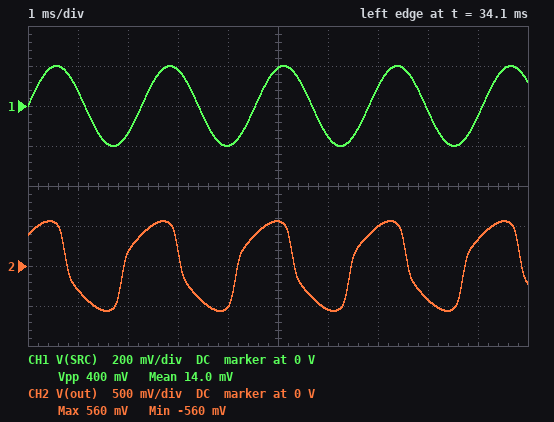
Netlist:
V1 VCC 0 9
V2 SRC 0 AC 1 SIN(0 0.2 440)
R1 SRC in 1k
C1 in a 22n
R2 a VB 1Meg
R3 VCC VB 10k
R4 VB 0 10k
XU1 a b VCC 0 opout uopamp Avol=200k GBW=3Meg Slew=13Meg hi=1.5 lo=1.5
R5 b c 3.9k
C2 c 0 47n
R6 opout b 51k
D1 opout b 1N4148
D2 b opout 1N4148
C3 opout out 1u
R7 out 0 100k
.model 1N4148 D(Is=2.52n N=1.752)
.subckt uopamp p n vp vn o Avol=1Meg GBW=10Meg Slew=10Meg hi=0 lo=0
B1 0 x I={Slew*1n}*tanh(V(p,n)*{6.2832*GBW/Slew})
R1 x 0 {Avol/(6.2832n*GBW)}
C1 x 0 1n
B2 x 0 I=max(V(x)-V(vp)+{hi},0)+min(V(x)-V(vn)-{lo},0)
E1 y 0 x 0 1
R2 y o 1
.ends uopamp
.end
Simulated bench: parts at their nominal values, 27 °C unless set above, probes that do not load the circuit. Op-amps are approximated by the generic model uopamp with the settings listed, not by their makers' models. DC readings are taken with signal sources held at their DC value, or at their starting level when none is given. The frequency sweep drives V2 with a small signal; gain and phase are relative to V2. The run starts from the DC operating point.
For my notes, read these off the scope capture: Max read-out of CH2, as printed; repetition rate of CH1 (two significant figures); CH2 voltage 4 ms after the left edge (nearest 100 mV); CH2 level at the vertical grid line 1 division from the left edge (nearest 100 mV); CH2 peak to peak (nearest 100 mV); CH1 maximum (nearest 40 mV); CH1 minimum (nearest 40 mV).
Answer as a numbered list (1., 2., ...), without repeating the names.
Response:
1. 560 mV
2. 440 Hz
3. -500 mV
4. -300 mV
5. 1.1 V
6. 200 mV
7. -200 mV
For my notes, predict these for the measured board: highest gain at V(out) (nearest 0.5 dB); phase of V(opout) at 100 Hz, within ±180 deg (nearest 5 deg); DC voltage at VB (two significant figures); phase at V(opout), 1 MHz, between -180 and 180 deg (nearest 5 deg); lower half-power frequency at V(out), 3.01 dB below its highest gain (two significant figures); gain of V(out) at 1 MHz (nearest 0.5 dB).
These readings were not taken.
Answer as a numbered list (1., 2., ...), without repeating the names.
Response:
1. 23.0 dB
2. 55 deg
3. 4.5 V
4. -80 deg
5. 860 Hz
6. 9.5 dB
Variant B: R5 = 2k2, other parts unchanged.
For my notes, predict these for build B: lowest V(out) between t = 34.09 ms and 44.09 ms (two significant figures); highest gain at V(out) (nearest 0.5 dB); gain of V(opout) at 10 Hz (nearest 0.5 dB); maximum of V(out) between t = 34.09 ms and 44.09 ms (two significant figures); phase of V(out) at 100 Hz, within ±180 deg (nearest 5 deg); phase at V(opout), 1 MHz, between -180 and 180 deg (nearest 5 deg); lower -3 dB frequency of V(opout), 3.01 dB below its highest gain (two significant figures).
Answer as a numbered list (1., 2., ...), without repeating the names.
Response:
1. -550 mV
2. 27.5 dB
3. -1.5 dB
4. 550 mV
5. 60 deg
6. -85 deg
7. 1.5 kHz
